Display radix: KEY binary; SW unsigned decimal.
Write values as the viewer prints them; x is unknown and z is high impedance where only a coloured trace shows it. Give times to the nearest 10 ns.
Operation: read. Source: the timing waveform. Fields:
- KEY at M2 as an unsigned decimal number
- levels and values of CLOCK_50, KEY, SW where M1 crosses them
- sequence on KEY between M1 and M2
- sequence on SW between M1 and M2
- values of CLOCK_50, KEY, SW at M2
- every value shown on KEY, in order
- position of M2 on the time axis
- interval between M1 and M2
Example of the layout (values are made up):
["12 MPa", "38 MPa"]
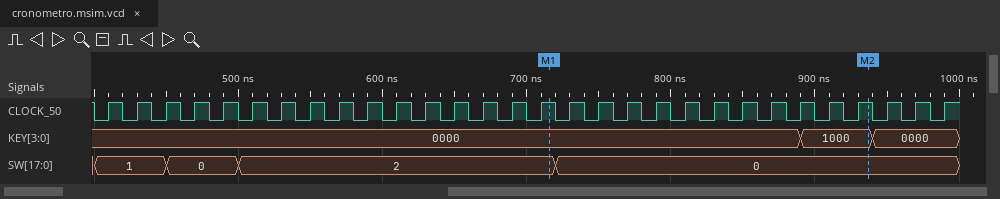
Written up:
["8", "CLOCK_50=1, KEY=0000, SW=2", "0000, 1000", "2, 0", "CLOCK_50=1, KEY=1000, SW=0", "0000, 1000, 0000", "940 ns", "220 ns"]
